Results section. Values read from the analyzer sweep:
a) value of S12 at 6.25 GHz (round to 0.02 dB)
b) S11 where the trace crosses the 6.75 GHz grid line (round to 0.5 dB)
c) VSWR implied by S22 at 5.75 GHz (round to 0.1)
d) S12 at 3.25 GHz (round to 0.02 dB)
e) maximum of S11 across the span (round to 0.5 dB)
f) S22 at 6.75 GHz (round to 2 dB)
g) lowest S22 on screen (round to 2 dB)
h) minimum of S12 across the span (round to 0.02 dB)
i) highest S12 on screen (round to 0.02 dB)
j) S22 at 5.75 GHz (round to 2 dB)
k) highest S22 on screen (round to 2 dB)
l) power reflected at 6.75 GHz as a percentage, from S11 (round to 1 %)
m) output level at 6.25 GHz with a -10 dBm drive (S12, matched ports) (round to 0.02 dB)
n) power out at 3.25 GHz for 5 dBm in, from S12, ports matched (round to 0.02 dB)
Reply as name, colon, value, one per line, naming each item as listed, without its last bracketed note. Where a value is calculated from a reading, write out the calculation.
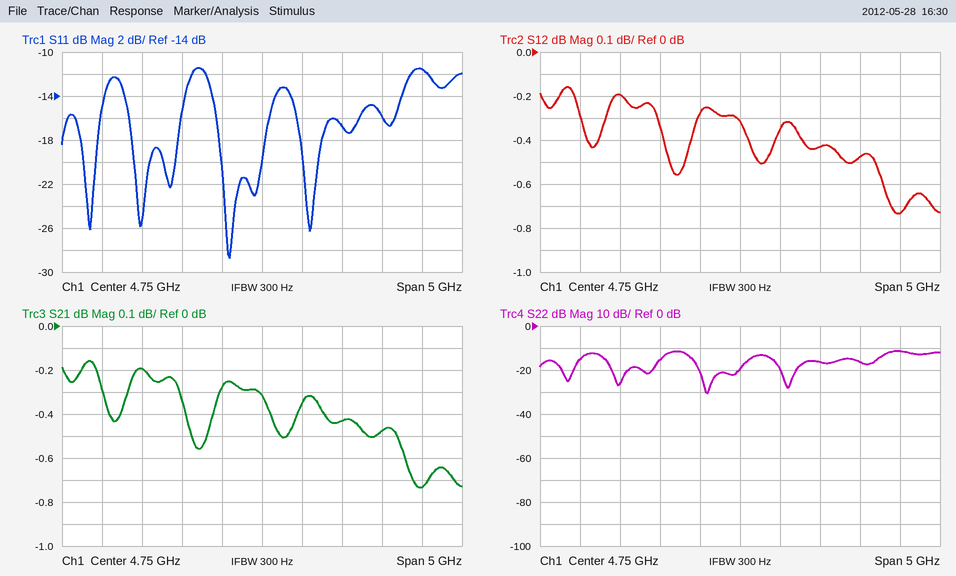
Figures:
value of S12 at 6.25 GHz: -0.48 dB
S11 where the trace crosses the 6.75 GHz grid line: -11.5 dB
VSWR implied by S22 at 5.75 GHz: |Γ| = 10^(-16/20) = 0.1585; VSWR = (1 + 0.1585)/(1 − 0.1585) ≈ 1.4
S12 at 3.25 GHz: -0.20 dB
maximum of S11 across the span: -11.5 dB
S22 at 6.75 GHz: -12 dB
lowest S22 on screen: -30 dB
minimum of S12 across the span: -0.74 dB
highest S12 on screen: -0.16 dB
S22 at 5.75 GHz: -16 dB
highest S22 on screen: -12 dB
power reflected at 6.75 GHz as a percentage, from S11: 10^(-11.5/10) ≈ 7 %
output level at 6.25 GHz with a -10 dBm drive (S12, matched ports): -10 dBm + (-0.48 dB) = -10.48 dBm
power out at 3.25 GHz for 5 dBm in, from S12, ports matched: 5 dBm + (-0.20 dB) = 4.80 dBm
